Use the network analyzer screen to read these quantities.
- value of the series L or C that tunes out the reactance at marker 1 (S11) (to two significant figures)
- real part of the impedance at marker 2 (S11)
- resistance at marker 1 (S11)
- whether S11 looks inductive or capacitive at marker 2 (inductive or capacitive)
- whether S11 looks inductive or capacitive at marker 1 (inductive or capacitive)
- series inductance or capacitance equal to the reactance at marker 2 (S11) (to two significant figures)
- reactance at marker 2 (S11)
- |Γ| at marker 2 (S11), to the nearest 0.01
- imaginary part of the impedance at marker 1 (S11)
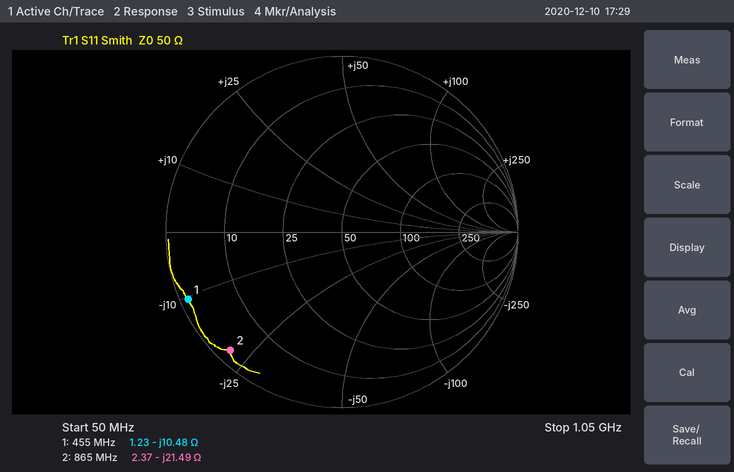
3.7 nH
2.37 Ω
1.23 Ω
capacitive
capacitive
8.6 pF
-21.49 Ω
0.92
-10.48 Ω
